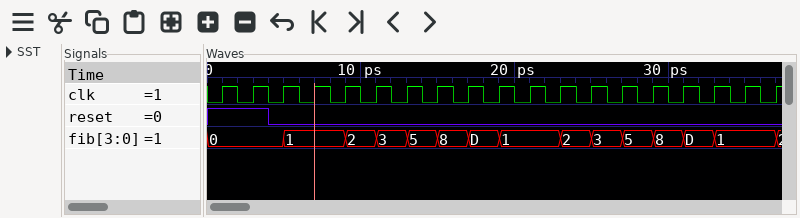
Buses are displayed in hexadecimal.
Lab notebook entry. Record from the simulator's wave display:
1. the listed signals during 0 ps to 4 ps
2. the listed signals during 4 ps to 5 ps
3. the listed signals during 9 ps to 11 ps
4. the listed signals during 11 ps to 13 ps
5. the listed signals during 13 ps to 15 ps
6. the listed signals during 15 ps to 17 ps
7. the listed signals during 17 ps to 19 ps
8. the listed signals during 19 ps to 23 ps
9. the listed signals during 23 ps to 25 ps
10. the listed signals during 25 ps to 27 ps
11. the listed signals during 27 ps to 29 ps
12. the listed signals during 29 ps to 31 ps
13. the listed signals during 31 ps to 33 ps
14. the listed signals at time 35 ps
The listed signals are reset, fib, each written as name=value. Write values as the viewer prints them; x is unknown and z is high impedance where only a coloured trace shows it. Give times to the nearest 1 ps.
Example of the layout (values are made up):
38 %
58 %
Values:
reset=1, fib=0
reset=0, fib=0
reset=0, fib=2
reset=0, fib=3
reset=0, fib=5
reset=0, fib=8
reset=0, fib=D
reset=0, fib=1
reset=0, fib=2
reset=0, fib=3
reset=0, fib=5
reset=0, fib=8
reset=0, fib=D
reset=0, fib=1
